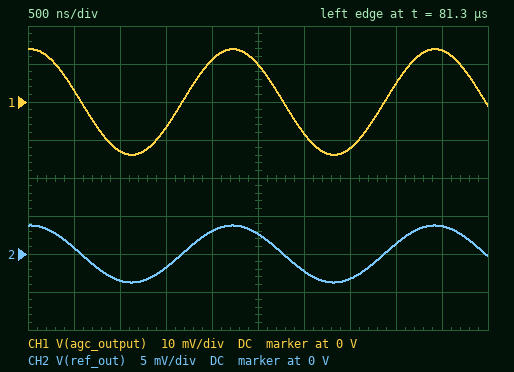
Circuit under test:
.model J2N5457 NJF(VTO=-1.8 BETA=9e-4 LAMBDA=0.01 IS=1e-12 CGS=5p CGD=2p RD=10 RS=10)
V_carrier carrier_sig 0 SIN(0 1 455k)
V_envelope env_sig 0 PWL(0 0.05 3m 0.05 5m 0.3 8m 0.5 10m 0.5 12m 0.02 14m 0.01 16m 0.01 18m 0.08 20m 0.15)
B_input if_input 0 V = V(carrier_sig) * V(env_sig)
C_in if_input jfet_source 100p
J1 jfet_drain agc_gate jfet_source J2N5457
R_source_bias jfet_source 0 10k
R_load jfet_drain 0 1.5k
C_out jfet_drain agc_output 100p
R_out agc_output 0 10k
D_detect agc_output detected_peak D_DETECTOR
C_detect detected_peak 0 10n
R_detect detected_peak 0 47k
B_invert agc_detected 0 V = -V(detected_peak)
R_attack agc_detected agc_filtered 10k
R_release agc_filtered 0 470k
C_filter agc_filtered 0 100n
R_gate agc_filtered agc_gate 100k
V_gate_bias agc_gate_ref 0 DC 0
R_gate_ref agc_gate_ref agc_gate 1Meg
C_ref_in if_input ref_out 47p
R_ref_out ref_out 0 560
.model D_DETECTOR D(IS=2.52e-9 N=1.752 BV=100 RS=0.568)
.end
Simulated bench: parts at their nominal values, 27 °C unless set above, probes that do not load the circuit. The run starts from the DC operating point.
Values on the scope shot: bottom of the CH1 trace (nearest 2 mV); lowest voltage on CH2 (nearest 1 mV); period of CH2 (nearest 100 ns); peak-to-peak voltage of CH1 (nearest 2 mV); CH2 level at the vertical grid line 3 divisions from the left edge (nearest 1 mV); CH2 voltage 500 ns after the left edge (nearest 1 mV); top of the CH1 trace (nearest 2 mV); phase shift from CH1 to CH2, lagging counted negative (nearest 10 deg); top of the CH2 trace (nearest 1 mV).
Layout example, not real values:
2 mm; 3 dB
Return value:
-14 mV; -4 mV; 2.2 µs; 28 mV; -2 mV; 1 mV; 14 mV; 0 deg; 4 mV
